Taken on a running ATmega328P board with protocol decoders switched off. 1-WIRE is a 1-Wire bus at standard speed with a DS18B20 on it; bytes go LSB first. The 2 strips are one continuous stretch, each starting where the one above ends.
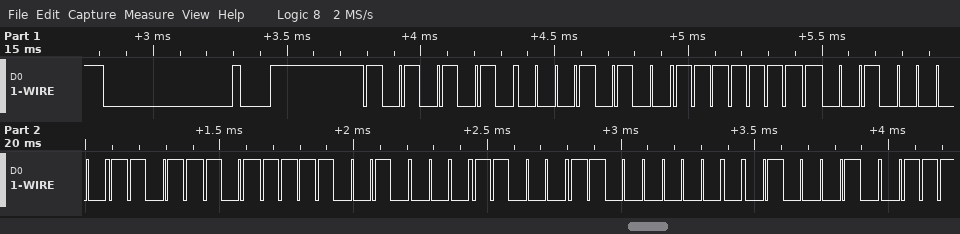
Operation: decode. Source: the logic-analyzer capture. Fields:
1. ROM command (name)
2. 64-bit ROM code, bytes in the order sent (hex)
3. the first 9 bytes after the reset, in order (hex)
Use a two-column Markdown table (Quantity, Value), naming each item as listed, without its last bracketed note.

| Quantity | Value |
|---|---|
| ROM command | Match ROM |
| 64-bit ROM code, bytes in the order sent | 28 FF 04 BB 4F 18 03 44 |
| the first 9 bytes after the reset, in order | 55 28 FF 04 BB 4F 18 03 44 |
